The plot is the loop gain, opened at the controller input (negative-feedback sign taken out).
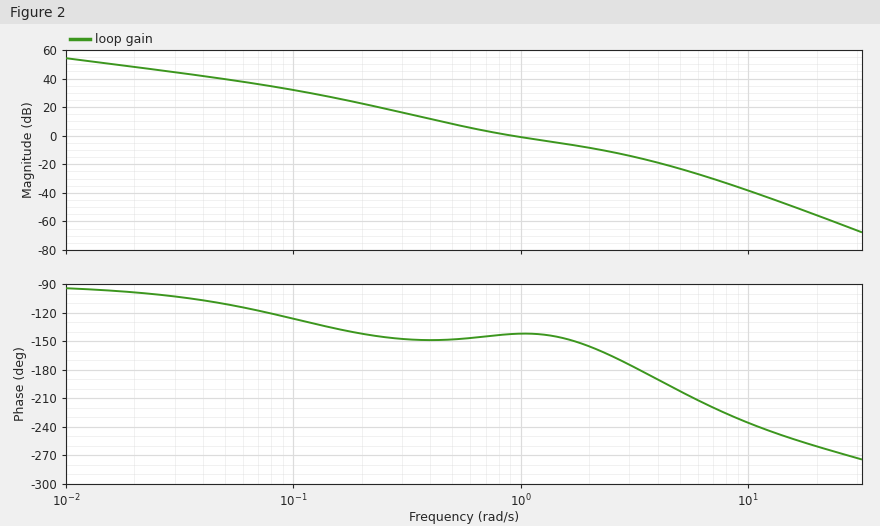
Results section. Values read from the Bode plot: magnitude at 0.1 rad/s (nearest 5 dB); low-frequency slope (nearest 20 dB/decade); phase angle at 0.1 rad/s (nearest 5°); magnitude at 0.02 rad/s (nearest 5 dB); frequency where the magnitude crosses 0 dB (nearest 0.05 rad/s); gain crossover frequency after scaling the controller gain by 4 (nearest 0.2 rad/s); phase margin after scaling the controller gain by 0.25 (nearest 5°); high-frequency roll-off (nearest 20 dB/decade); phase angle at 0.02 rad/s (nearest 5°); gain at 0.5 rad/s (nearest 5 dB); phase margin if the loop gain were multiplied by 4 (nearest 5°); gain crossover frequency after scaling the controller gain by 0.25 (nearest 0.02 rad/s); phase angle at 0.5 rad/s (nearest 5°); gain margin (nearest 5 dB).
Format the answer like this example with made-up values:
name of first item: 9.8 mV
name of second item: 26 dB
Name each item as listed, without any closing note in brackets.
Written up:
magnitude at 0.1 rad/s: 30 dB
low-frequency slope: -20 dB/decade
phase angle at 0.1 rad/s: -125°
magnitude at 0.02 rad/s: 50 dB
frequency where the magnitude crosses 0 dB: 0.90 rad/s
gain crossover frequency after scaling the controller gain by 4: 2.6 rad/s
phase margin after scaling the controller gain by 0.25: 30°
high-frequency roll-off: -60 dB/decade
phase angle at 0.02 rad/s: -100°
gain at 0.5 rad/s: 10 dB
phase margin if the loop gain were multiplied by 4: 10°
gain crossover frequency after scaling the controller gain by 0.25: 0.40 rad/s
phase angle at 0.5 rad/s: -150°
gain margin: 15 dB
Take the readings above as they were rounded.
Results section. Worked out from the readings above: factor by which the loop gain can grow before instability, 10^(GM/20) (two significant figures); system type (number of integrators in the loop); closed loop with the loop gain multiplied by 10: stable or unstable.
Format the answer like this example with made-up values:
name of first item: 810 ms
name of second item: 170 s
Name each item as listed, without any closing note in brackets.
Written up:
factor by which the loop gain can grow before instability, 10^(GM/20): 5.6
system type: 1
closed loop with the loop gain multiplied by 10: stable or unstable: unstable
